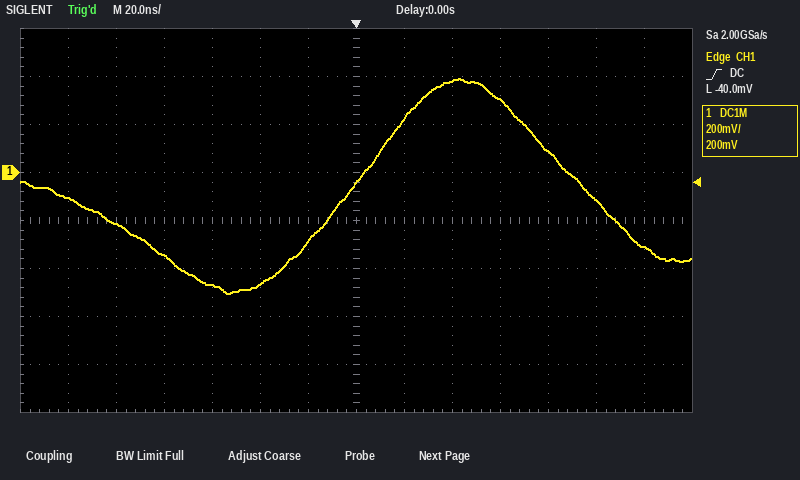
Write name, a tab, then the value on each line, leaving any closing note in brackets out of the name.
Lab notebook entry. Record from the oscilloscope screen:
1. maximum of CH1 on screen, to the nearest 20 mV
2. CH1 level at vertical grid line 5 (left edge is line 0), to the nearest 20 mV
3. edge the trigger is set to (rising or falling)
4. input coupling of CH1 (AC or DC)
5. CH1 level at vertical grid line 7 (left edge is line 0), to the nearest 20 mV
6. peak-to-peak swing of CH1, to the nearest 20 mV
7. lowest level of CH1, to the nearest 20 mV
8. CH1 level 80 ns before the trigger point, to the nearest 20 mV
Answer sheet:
maximum of CH1 on screen, to the nearest 20 mV	400 mV
CH1 level at vertical grid line 5 (left edge is line 0), to the nearest 20 mV	-460 mV
edge the trigger is set to	rising
input coupling of CH1	DC
CH1 level at vertical grid line 7 (left edge is line 0), to the nearest 20 mV	-40 mV
peak-to-peak swing of CH1, to the nearest 20 mV	900 mV
lowest level of CH1, to the nearest 20 mV	-500 mV
CH1 level 80 ns before the trigger point, to the nearest 20 mV	-340 mV
